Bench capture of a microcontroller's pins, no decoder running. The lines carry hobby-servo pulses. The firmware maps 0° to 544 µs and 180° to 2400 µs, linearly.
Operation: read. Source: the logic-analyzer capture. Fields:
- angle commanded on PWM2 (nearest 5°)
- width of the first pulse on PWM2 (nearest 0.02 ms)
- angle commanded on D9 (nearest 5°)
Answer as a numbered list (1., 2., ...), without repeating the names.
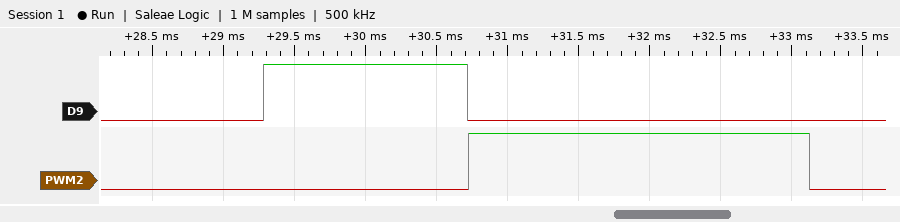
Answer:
1. 180°
2. 2.40 ms
3. 85°
